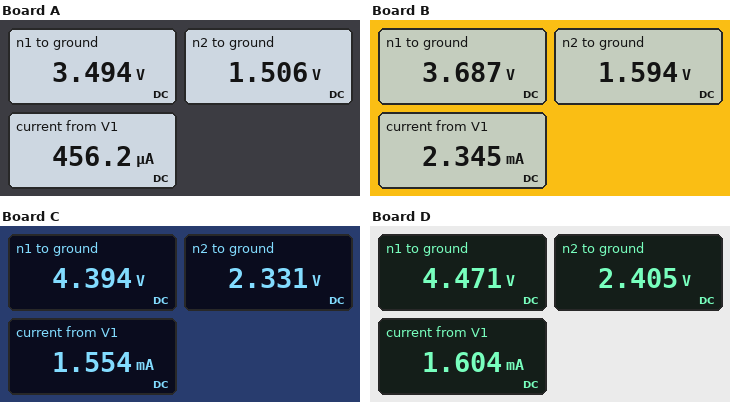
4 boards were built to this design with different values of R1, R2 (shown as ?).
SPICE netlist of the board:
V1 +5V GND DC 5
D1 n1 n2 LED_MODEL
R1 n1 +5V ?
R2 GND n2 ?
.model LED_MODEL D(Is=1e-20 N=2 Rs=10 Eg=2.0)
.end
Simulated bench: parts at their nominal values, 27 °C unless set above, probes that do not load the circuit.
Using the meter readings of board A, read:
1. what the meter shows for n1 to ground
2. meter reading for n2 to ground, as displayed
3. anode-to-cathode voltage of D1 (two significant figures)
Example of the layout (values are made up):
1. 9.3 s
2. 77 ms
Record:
1. 3.494 V
2. 1.506 V
3. 2.0 V
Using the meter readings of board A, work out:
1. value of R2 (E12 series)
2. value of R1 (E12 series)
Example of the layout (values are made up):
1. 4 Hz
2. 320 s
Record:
1. 3.3 kΩ
2. 3.3 kΩ
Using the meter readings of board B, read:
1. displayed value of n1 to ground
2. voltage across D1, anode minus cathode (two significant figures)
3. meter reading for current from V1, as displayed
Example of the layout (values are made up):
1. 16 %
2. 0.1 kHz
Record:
1. 3.687 V
2. 2.1 V
3. 2.345 mA
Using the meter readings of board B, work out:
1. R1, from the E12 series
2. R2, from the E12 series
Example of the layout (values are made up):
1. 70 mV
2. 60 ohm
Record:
1. 560 Ω
2. 680 Ω
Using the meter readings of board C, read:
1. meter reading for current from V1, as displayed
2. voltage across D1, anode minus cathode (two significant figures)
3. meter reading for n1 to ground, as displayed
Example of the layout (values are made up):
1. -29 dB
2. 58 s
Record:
1. 1.554 mA
2. 2.1 V
3. 4.394 V
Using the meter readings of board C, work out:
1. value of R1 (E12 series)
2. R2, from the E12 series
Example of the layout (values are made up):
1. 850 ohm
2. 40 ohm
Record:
1. 390 Ω
2. 1.5 kΩ
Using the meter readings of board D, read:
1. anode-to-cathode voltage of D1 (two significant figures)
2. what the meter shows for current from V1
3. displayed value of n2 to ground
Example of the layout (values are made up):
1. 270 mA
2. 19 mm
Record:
1. 2.1 V
2. 1.604 mA
3. 2.405 V
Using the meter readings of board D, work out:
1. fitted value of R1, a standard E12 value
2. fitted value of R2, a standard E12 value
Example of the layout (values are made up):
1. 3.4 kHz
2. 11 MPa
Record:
1. 330 Ω
2. 1.5 kΩ
